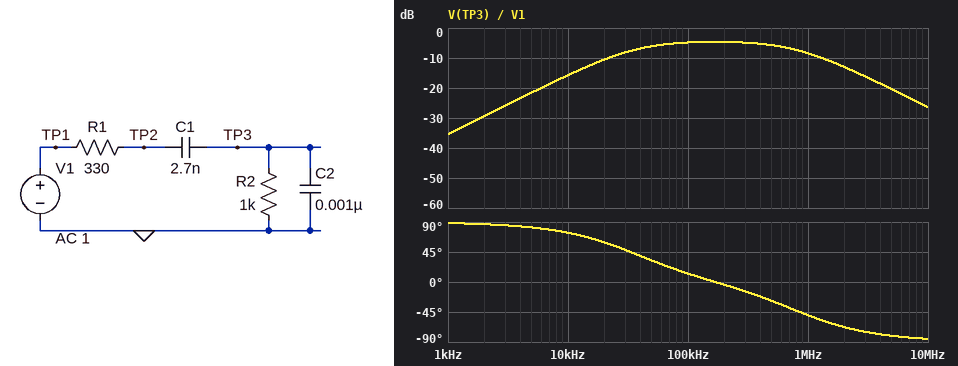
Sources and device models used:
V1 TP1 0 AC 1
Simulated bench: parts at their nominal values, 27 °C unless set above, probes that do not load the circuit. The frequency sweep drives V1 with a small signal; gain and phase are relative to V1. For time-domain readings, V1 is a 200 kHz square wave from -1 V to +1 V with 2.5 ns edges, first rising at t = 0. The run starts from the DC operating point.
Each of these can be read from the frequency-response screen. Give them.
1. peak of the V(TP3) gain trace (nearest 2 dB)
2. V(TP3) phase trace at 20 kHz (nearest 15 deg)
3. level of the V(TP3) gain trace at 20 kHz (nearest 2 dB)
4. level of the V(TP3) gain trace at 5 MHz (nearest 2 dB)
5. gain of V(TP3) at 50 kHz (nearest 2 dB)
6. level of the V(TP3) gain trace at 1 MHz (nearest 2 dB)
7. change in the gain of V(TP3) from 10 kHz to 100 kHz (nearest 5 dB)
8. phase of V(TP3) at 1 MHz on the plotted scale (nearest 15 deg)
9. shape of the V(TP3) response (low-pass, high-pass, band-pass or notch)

-4 dB
60 deg
-10 dB
-20 dB
-6 dB
-8 dB
10 dB
-45 deg
band-pass
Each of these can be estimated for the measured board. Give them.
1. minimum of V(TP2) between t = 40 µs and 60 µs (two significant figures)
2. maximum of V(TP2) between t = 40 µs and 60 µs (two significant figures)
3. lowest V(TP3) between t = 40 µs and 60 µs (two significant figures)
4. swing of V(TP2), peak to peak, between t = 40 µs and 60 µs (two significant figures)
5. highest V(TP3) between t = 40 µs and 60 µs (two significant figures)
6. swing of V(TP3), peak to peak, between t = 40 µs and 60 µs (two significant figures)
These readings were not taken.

-880 mV
880 mV
-660 mV
1.8 V
660 mV
1.3 V
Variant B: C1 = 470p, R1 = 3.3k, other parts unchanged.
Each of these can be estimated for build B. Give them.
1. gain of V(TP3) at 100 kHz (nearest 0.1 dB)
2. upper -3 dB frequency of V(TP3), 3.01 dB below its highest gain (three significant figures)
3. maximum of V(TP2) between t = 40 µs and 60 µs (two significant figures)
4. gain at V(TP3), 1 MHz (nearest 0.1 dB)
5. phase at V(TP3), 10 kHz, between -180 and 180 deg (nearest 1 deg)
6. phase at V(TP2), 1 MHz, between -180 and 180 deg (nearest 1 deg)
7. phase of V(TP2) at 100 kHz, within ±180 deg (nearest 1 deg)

-16.3 dB
356 kHz
710 mV
-26.6 dB
79 deg
-79 deg
-36 deg
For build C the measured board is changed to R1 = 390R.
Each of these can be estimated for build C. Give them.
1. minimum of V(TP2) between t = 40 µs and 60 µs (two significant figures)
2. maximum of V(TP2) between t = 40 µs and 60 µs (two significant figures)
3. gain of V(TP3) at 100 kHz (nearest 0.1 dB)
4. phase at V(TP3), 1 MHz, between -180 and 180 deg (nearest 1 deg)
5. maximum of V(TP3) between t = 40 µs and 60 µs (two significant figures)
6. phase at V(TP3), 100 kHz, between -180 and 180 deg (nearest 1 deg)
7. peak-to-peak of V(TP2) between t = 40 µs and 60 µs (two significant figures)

-860 mV
860 mV
-5.1 dB
-54 deg
630 mV
11 deg
1.7 V
